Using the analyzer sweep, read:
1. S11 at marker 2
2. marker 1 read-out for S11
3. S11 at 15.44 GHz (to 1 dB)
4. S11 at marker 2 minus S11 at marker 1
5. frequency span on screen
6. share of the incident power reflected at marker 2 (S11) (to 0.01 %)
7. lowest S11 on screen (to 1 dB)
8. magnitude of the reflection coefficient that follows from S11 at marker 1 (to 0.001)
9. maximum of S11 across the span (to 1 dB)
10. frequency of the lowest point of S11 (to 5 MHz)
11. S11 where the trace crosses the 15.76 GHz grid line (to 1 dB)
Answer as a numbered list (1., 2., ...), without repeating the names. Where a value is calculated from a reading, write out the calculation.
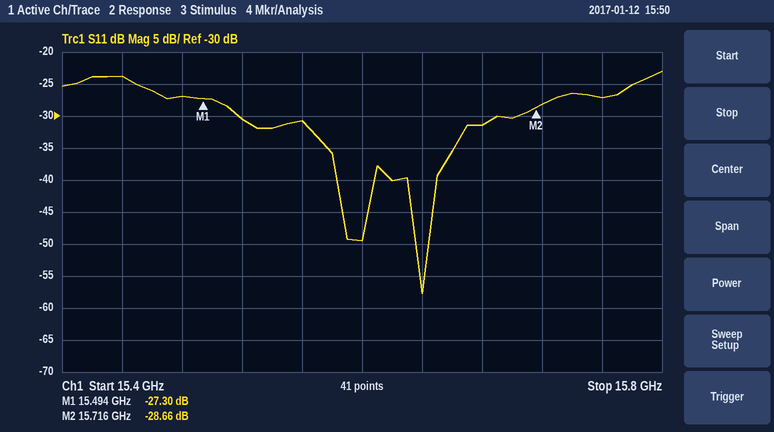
1. -28.66 dB
2. -27.30 dB
3. -24 dB
4. -28.66 − (-27.3) = -1.36 dB
5. 400 MHz
6. 10^(-28.66/10) ≈ 0.14 %
7. -58 dB
8. 10^(-27.3/20) ≈ 0.043
9. -23 dB
10. 15.640 GHz
11. -27 dB
